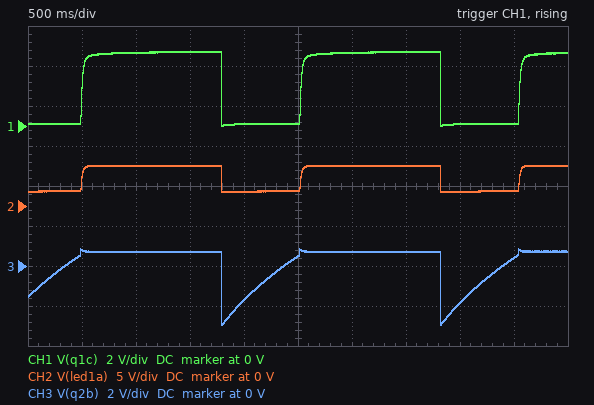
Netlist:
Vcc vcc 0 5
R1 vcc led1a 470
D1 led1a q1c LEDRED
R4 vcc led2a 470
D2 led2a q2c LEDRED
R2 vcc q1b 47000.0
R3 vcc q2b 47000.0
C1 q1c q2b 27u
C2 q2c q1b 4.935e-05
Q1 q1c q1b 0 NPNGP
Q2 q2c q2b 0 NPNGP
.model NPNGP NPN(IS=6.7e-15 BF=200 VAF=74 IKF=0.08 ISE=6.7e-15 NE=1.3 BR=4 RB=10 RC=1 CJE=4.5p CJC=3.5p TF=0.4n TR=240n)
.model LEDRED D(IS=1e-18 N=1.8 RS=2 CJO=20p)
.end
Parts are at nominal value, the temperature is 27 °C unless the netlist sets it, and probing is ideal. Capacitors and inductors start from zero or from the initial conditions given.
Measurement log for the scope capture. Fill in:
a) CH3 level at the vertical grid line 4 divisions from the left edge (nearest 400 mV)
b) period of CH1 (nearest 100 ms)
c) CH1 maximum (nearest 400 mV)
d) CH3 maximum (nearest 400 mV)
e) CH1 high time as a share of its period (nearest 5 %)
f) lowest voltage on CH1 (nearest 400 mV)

-1.6 V
2.0 s
3.6 V
800 mV
65 %
0 V
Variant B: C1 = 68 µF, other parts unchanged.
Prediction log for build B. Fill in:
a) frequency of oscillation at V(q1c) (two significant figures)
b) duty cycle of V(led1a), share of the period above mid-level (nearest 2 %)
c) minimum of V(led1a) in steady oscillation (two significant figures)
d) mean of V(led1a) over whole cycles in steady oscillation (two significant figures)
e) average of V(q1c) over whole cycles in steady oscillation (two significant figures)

320 mHz
42 %
1.7 V
3.1 V
1.5 V
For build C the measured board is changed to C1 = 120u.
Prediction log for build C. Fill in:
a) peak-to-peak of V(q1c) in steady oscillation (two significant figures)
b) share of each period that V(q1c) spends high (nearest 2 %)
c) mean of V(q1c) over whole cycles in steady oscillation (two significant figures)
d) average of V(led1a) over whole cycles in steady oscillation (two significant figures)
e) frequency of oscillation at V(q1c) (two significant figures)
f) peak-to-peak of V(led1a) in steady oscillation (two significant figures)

3.6 V
28 %
1.1 V
2.7 V
220 mHz
3.3 V
